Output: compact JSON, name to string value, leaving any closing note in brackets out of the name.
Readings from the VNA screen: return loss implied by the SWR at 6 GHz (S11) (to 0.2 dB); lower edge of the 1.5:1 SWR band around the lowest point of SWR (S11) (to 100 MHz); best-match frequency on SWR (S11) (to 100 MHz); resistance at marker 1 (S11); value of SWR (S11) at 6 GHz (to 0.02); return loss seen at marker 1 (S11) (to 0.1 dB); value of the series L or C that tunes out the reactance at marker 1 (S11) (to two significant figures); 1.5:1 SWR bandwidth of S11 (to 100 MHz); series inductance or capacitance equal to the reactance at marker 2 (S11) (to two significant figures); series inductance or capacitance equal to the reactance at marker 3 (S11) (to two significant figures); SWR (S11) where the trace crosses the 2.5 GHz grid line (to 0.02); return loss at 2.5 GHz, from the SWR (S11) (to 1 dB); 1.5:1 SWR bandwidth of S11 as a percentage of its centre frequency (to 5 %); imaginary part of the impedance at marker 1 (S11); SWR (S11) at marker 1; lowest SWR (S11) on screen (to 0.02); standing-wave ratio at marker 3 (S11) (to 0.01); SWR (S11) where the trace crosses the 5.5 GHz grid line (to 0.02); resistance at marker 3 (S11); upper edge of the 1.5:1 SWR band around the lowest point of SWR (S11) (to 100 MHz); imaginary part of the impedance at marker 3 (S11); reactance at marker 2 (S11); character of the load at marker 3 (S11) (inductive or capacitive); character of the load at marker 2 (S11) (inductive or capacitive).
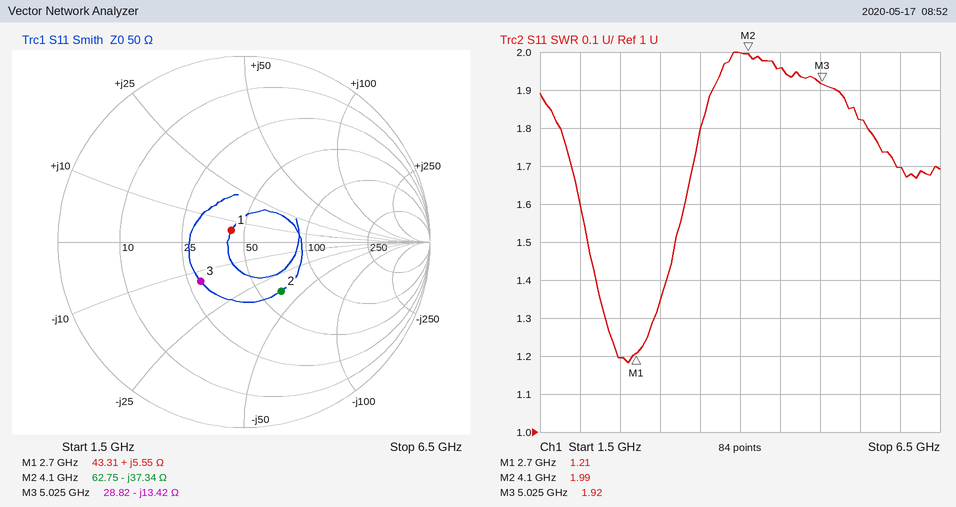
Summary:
{"return loss implied by the SWR at 6 GHz (S11)": "11.8 dB", "lower edge of the 1.5:1 SWR band around the lowest point of SWR (S11)": "2.1 GHz", "best-match frequency on SWR (S11)": "2.6 GHz", "resistance at marker 1": "43.31 Ω", "value of SWR (S11) at 6 GHz": "1.70", "return loss seen at marker 1 (S11)": "20.6 dB", "value of the series L or C that tunes out the reactance at marker 1 (S11)": "11 pF", "1.5:1 SWR bandwidth of S11": "1.1 GHz", "series inductance or capacitance equal to the reactance at marker 2 (S11)": "1.0 pF", "series inductance or capacitance equal to the reactance at marker 3 (S11)": "2.4 pF", "SWR (S11) where the trace crosses the 2.5 GHz grid line": "1.20", "return loss at 2.5 GHz, from the SWR (S11)": "21 dB", "1.5:1 SWR bandwidth of S11 as a percentage of its centre frequency": "40 %", "imaginary part of the impedance at marker 1": "+5.55 Ω", "SWR (S11) at marker 1": "1.21", "lowest SWR (S11) on screen": "1.18", "standing-wave ratio at marker 3 (S11)": "1.91", "SWR (S11) where the trace crosses the 5.5 GHz grid line": "1.82", "resistance at marker 3": "28.82 Ω", "upper edge of the 1.5:1 SWR band around the lowest point of SWR (S11)": "3.2 GHz", "imaginary part of the impedance at marker 3": "-13.42 Ω", "reactance at marker 2": "-37.34 Ω", "character of the load at marker 3 (S11)": "capacitive", "character of the load at marker 2 (S11)": "capacitive"}
